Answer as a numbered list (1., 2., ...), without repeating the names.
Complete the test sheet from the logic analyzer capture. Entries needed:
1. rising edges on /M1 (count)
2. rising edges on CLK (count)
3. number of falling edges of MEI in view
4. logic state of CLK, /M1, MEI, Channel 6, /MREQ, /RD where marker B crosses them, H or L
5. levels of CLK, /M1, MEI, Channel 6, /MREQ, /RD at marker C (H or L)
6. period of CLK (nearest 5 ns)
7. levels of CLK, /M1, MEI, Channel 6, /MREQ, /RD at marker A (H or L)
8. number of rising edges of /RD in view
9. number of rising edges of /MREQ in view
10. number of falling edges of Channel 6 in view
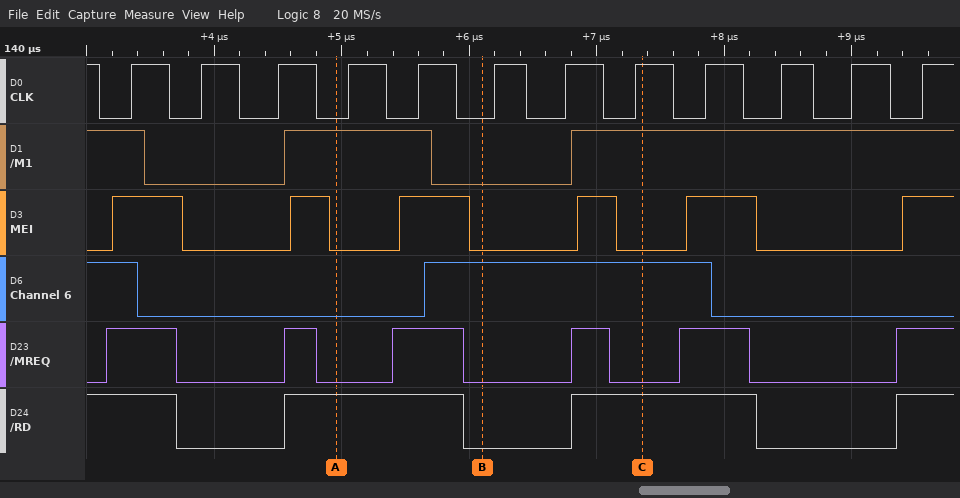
1. 2
2. 12
3. 5
4. CLK=L, /M1=L, MEI=L, Channel 6=H, /MREQ=L, /RD=L
5. CLK=H, /M1=H, MEI=L, Channel 6=H, /MREQ=L, /RD=H
6. 565 ns
7. CLK=L, /M1=H, MEI=L, Channel 6=L, /MREQ=L, /RD=H
8. 3
9. 6
10. 2
